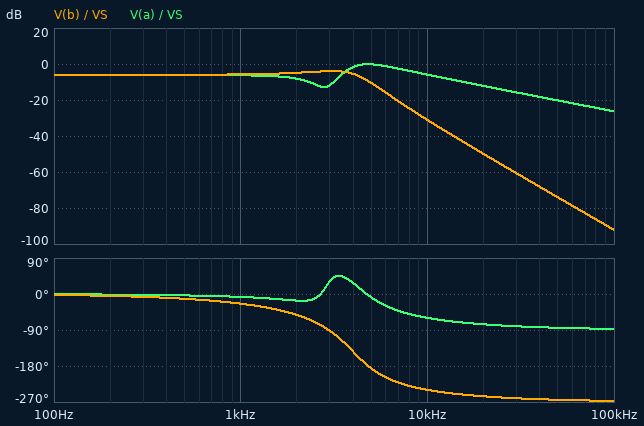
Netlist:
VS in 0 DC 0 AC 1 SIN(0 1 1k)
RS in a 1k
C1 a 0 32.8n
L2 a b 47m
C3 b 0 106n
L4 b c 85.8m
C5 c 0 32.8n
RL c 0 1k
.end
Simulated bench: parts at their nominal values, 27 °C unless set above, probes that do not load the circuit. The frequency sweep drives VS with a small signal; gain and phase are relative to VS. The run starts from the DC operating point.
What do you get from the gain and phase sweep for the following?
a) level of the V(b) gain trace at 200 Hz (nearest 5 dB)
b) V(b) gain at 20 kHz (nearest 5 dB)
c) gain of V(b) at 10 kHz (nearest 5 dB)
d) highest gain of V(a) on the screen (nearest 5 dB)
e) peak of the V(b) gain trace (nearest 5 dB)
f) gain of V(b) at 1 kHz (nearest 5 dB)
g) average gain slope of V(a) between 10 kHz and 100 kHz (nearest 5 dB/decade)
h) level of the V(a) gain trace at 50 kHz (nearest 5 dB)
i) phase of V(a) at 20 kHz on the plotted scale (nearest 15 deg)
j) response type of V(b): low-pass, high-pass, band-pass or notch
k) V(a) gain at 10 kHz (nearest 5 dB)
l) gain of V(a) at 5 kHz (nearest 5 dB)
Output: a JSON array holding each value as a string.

["-5 dB", "-50 dB", "-30 dB", "0 dB", "-5 dB", "-5 dB", "-20 dB/decade", "-20 dB", "-75 deg", "low-pass", "-5 dB", "0 dB"]
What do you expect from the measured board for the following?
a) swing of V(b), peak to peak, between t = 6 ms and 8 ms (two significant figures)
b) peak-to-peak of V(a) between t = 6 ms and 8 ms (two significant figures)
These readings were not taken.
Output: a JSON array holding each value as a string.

["1.0 V", "970 mV"]
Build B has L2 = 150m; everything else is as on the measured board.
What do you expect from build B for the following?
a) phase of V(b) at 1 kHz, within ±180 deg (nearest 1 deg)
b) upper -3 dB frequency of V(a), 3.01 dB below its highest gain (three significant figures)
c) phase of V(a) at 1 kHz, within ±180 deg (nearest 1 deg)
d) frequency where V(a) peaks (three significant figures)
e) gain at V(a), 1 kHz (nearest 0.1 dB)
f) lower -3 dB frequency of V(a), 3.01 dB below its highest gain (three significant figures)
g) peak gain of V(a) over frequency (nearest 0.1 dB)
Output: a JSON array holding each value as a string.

["-43 deg", "6.20 kHz", "9 deg", "3.09 kHz", "-5.0 dB", "1.81 kHz", "-0.4 dB"]
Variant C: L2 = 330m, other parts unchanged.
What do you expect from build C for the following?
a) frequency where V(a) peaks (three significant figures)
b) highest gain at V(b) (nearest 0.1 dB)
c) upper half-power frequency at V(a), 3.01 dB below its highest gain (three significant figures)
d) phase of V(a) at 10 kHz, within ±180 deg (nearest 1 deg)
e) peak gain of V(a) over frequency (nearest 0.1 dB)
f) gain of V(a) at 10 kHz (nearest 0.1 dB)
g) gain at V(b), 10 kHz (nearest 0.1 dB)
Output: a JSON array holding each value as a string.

["2.27 kHz", "-6.0 dB", "5.79 kHz", "-64 deg", "-0.5 dB", "-7.0 dB", "-49.5 dB"]
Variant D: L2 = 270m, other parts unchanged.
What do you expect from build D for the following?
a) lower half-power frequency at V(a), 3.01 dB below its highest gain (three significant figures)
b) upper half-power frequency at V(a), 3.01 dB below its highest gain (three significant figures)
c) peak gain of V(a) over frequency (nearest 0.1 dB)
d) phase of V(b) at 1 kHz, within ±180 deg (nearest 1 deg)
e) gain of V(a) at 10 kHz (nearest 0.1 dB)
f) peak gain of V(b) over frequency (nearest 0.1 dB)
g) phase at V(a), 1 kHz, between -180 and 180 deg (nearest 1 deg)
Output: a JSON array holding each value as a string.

["806 Hz", "5.89 kHz", "-0.5 dB", "-63 deg", "-7.0 dB", "-6.0 dB", "12 deg"]
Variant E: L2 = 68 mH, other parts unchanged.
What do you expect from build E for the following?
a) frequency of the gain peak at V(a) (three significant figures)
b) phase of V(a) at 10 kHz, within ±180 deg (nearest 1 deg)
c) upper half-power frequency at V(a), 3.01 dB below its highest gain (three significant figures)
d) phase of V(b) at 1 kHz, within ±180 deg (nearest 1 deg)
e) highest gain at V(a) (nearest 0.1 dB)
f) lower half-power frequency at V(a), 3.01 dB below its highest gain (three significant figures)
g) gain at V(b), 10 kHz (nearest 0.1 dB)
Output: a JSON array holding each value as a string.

["4.12 kHz", "-61 deg", "6.88 kHz", "-28 deg", "-0.2 dB", "3.16 kHz", "-34.8 dB"]
